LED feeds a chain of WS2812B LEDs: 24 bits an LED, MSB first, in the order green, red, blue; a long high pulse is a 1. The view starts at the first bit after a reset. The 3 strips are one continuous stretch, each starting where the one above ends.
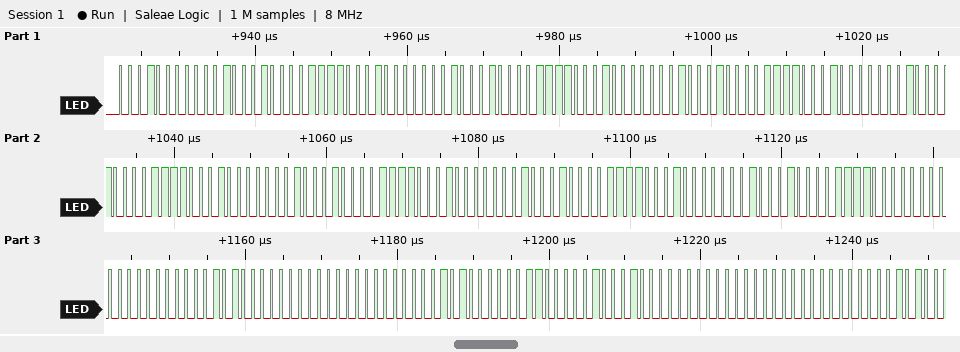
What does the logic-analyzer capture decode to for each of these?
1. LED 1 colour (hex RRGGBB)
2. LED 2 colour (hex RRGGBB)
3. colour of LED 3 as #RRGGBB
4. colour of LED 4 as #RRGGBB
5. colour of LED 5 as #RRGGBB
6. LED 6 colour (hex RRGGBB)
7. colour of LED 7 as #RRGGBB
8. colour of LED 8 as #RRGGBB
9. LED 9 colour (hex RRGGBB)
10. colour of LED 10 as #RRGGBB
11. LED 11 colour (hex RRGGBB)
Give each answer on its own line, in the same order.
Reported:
#11100F
#11100F
#11100F
#11100F
#11100F
#11100F
#11100F
#000014
#000014
#110C00
#000014
